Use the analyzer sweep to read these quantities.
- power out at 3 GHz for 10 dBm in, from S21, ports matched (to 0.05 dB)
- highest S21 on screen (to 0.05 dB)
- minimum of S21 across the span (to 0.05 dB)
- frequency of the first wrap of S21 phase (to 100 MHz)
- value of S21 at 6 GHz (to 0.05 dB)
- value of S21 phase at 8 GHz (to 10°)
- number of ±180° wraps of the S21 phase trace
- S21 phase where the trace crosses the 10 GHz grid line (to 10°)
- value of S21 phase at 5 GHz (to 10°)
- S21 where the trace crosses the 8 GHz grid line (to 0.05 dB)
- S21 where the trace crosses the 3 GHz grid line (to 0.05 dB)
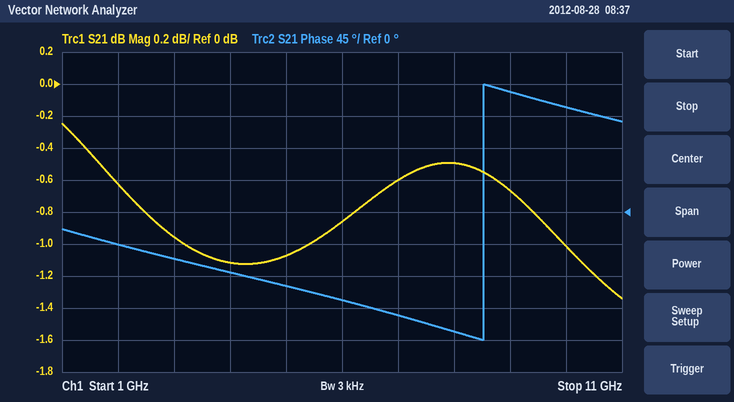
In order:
9.05 dBm
-0.25 dB
-1.35 dB
8.5 GHz
-0.85 dB
-170°
1
150°
-100°
-0.50 dB
-0.95 dB
